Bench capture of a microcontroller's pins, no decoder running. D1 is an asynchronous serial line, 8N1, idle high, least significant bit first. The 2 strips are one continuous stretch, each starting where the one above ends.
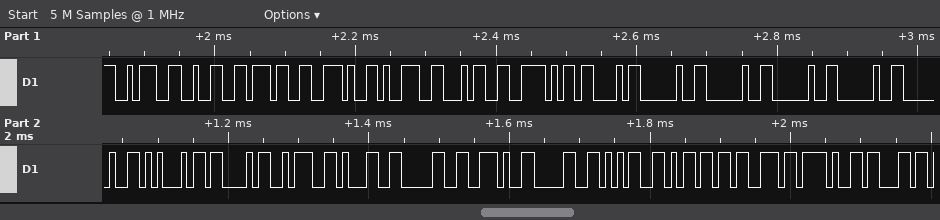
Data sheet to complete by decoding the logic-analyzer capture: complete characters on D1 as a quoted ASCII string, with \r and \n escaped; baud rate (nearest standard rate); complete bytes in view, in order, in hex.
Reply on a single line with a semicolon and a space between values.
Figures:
":27.94^C     EC:10.05ms/c"; 115200 baud; 3A 32 37 2E 39 34 5E 43 20 20 20 20 20 45 43 3A 31 30 2E 30 35 6D 73 2F 63
